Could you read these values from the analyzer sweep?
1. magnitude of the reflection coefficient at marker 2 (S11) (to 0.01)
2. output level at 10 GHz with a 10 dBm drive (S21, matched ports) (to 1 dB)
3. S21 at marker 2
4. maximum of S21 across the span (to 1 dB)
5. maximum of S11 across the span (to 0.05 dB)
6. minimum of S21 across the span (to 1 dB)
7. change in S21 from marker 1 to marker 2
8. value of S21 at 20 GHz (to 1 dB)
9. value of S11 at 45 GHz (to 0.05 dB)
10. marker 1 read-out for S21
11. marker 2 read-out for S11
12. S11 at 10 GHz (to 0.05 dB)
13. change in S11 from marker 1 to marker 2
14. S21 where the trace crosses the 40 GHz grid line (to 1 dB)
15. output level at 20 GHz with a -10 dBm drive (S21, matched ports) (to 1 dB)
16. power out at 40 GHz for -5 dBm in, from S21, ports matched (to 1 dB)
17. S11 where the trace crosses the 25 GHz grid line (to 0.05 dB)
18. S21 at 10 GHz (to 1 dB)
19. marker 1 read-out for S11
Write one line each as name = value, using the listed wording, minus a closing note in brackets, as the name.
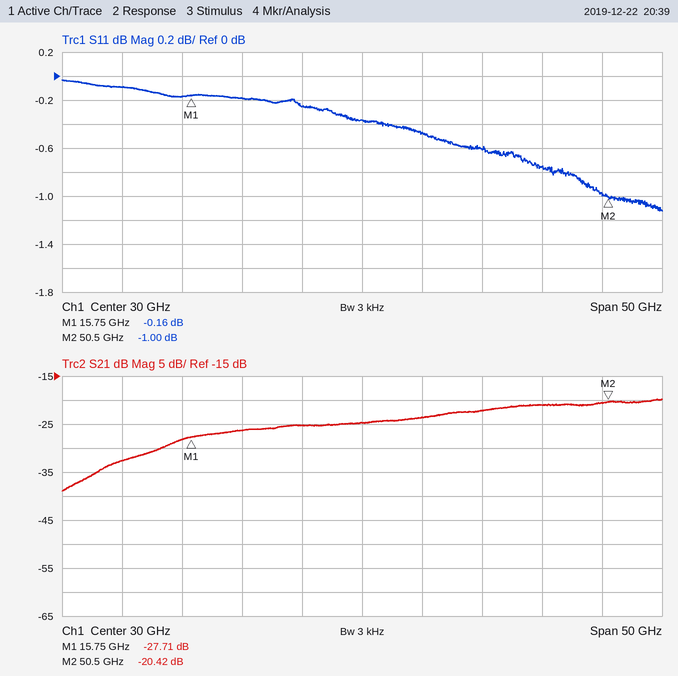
magnitude of the reflection coefficient at marker 2 (S11) = 0.89
output level at 10 GHz with a 10 dBm drive (S21, matched ports) = -23 dBm
S21 at marker 2 = -20.42 dB
maximum of S21 across the span = -20 dB
maximum of S11 across the span = -0.05 dB
minimum of S21 across the span = -39 dB
change in S21 from marker 1 to marker 2 = 7.29 dB
value of S21 at 20 GHz = -26 dB
value of S11 at 45 GHz = -0.75 dB
marker 1 read-out for S21 = -27.71 dB
marker 2 read-out for S11 = -1.00 dB
S11 at 10 GHz = -0.10 dB
change in S11 from marker 1 to marker 2 = -0.84 dB
S21 where the trace crosses the 40 GHz grid line = -22 dB
output level at 20 GHz with a -10 dBm drive (S21, matched ports) = -36 dBm
power out at 40 GHz for -5 dBm in, from S21, ports matched = -27 dBm
S11 where the trace crosses the 25 GHz grid line = -0.25 dB
S21 at 10 GHz = -33 dB
marker 1 read-out for S11 = -0.16 dB
